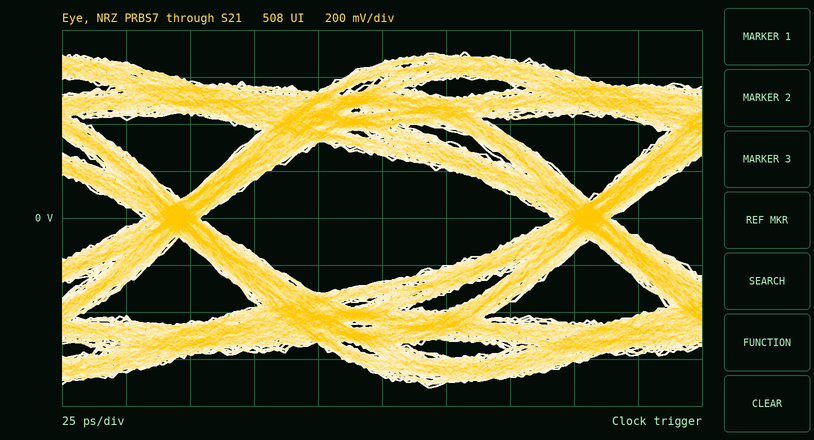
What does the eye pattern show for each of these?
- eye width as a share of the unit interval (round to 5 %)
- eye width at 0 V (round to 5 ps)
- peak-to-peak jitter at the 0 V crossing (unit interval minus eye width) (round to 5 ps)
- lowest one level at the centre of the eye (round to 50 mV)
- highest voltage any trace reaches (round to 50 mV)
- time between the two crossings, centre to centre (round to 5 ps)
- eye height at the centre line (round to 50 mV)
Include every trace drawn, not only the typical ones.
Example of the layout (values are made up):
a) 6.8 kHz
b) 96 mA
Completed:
a) 85 %
b) 140 ps
c) 20 ps
d) 250 mV
e) 700 mV
f) 160 ps
g) 550 mV
